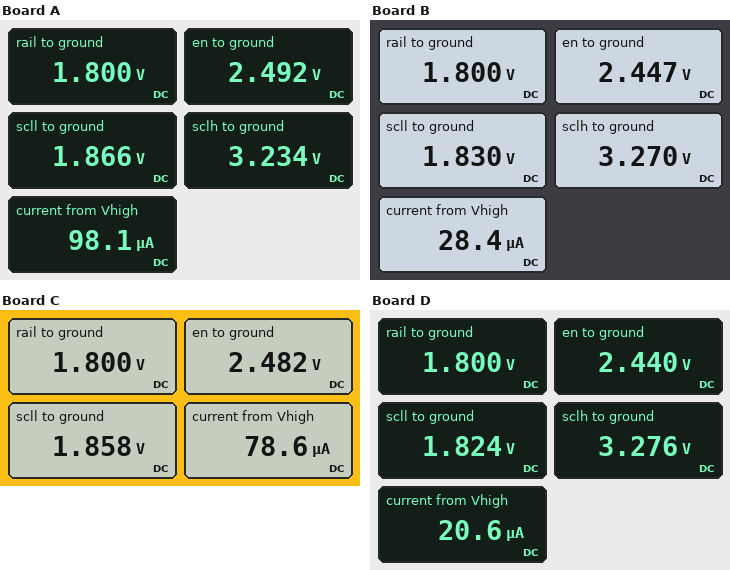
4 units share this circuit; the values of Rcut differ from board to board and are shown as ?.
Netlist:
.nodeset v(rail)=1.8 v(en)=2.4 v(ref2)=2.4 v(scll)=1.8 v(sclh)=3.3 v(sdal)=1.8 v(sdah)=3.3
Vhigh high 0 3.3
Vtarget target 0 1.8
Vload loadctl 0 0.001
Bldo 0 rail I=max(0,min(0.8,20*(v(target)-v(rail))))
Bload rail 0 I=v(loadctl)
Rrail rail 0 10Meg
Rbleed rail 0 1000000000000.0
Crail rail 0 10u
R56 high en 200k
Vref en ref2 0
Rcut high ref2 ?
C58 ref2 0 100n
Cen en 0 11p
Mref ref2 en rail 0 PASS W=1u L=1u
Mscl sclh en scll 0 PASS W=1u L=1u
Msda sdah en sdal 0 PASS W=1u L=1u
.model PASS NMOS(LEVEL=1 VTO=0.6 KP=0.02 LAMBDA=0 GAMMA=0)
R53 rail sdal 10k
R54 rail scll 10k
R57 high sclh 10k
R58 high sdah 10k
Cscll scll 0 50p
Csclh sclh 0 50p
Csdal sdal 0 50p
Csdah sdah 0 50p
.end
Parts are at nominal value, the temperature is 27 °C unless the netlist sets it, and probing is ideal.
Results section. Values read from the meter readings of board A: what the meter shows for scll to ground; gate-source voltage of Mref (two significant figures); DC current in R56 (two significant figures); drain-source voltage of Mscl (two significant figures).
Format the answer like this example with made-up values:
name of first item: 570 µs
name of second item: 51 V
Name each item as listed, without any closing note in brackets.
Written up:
what the meter shows for scll to ground: 1.866 V
gate-source voltage of Mref: 690 mV
DC current in R56: 4.0 µA
drain-source voltage of Mscl: 1.4 V
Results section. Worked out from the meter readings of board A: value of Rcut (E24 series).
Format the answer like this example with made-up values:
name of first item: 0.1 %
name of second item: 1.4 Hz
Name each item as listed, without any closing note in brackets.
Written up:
value of Rcut: 10 kΩ
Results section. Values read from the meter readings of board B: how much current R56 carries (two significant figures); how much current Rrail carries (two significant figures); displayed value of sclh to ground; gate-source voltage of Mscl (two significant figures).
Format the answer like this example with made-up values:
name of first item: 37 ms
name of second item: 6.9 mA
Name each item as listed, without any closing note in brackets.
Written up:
how much current R56 carries: 4.3 µA
how much current Rrail carries: 180 nA
displayed value of sclh to ground: 3.270 V
gate-source voltage of Mscl: 620 mV
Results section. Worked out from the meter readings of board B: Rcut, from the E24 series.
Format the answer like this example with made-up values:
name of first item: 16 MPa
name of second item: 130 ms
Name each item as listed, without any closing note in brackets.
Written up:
Rcut, from the E24 series: 47 kΩ
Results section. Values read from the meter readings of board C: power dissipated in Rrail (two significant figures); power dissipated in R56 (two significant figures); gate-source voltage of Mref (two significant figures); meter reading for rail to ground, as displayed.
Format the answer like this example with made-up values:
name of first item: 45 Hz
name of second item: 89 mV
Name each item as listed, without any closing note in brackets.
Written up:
power dissipated in Rrail: 320 nW
power dissipated in R56: 3.3 µW
gate-source voltage of Mref: 680 mV
meter reading for rail to ground, as displayed: 1.800 V
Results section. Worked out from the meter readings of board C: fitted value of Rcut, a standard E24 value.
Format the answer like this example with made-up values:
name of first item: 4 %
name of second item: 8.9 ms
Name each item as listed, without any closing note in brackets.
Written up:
fitted value of Rcut, a standard E24 value: 13 kΩ
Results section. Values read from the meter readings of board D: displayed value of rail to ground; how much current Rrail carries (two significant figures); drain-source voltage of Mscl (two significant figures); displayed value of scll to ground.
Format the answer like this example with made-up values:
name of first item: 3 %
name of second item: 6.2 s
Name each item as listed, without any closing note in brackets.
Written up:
displayed value of rail to ground: 1.800 V
how much current Rrail carries: 180 nA
drain-source voltage of Mscl: 1.5 V
displayed value of scll to ground: 1.824 V
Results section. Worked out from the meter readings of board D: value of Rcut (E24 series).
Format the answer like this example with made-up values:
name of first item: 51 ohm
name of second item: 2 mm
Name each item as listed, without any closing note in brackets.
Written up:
value of Rcut: 75 kΩ
